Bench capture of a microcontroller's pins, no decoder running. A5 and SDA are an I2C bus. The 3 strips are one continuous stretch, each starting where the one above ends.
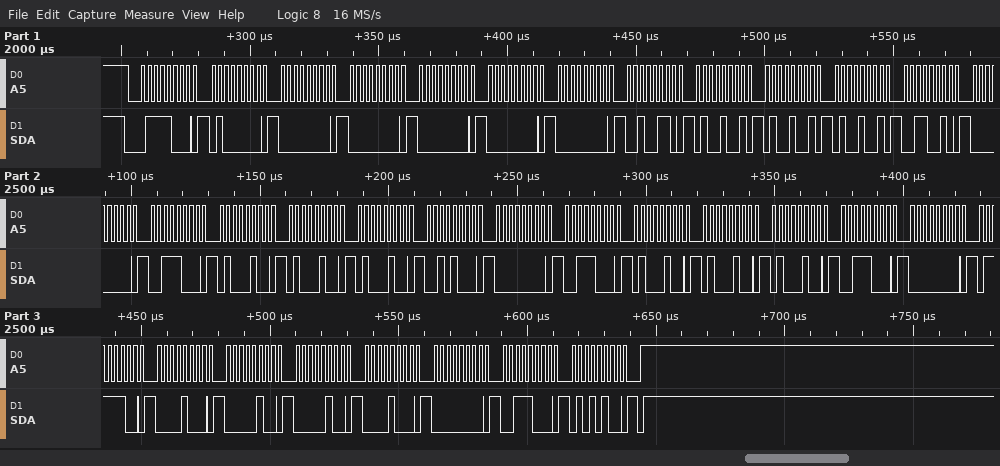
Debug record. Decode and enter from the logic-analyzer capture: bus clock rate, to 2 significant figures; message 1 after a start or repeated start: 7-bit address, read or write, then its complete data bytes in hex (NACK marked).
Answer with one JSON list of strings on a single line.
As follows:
["400 kHz", "0x3C write: 40 00 00 00 00 00 26 49 49 49 32 00 38 44 44 44 28 00 38 44 44 44 38 00 7C 08 04 04 08 00 38 54"]
